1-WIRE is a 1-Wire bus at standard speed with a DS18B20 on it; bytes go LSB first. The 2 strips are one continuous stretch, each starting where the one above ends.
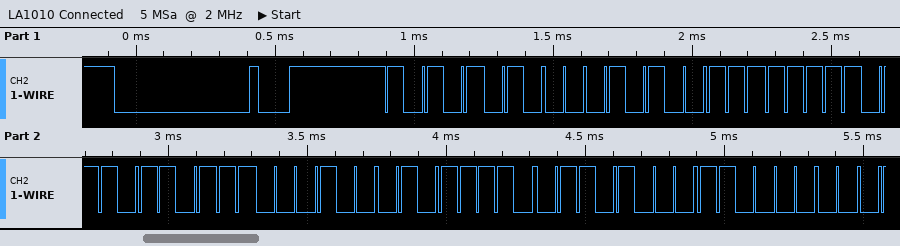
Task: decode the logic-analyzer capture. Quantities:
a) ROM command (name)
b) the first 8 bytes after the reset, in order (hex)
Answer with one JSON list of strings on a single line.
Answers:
["Match ROM", "55 28 FF B6 23 7A 16 03"]
